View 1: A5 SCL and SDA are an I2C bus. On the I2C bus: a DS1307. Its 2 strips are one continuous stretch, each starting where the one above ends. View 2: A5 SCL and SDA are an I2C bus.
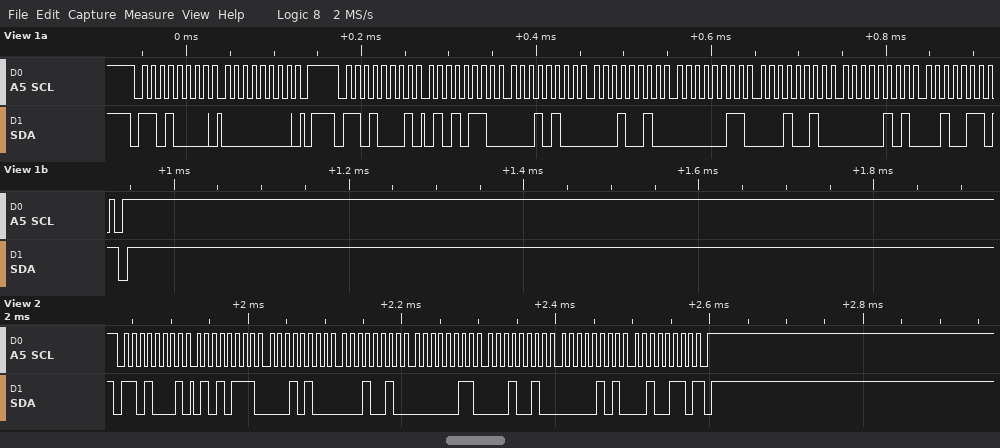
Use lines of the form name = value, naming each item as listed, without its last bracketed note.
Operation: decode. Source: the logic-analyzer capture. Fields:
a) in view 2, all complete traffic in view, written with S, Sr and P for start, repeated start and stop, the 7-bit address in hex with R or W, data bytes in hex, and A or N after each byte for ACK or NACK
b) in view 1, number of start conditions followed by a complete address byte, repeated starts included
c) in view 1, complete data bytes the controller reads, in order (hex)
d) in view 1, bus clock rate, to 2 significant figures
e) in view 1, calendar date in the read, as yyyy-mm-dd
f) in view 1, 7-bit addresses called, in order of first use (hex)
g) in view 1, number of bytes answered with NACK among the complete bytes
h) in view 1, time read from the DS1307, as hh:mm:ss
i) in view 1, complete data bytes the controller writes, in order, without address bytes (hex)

in view 2, all complete traffic in view, written with S, Sr and P for start, repeated start and stop, the 7-bit address in hex with R or W, data bytes in hex, and A or N after each byte for ACK or NACK = S 68R A 57 A 14 A 12 A 03 A 12 A 05 A 26 N P
in view 1, number of start conditions followed by a complete address byte, repeated starts included = 2
in view 1, complete data bytes the controller reads, in order = 56 14 12 03 12 05 26
in view 1, bus clock rate, to 2 significant figures = 100 kHz
in view 1, calendar date in the read, as yyyy-mm-dd = 2026-05-12
in view 1, 7-bit addresses called, in order of first use = 0x68
in view 1, number of bytes answered with NACK among the complete bytes = 1
in view 1, time read from the DS1307, as hh:mm:ss = 12:14:56
in view 1, complete data bytes the controller writes, in order, without address bytes = 00
